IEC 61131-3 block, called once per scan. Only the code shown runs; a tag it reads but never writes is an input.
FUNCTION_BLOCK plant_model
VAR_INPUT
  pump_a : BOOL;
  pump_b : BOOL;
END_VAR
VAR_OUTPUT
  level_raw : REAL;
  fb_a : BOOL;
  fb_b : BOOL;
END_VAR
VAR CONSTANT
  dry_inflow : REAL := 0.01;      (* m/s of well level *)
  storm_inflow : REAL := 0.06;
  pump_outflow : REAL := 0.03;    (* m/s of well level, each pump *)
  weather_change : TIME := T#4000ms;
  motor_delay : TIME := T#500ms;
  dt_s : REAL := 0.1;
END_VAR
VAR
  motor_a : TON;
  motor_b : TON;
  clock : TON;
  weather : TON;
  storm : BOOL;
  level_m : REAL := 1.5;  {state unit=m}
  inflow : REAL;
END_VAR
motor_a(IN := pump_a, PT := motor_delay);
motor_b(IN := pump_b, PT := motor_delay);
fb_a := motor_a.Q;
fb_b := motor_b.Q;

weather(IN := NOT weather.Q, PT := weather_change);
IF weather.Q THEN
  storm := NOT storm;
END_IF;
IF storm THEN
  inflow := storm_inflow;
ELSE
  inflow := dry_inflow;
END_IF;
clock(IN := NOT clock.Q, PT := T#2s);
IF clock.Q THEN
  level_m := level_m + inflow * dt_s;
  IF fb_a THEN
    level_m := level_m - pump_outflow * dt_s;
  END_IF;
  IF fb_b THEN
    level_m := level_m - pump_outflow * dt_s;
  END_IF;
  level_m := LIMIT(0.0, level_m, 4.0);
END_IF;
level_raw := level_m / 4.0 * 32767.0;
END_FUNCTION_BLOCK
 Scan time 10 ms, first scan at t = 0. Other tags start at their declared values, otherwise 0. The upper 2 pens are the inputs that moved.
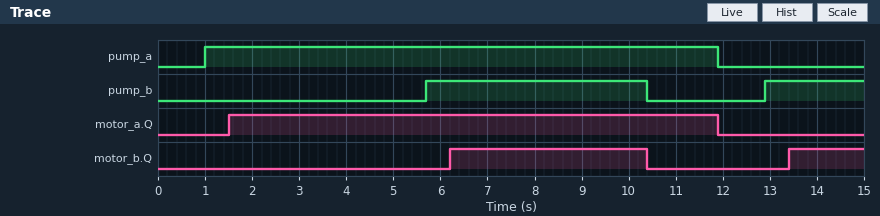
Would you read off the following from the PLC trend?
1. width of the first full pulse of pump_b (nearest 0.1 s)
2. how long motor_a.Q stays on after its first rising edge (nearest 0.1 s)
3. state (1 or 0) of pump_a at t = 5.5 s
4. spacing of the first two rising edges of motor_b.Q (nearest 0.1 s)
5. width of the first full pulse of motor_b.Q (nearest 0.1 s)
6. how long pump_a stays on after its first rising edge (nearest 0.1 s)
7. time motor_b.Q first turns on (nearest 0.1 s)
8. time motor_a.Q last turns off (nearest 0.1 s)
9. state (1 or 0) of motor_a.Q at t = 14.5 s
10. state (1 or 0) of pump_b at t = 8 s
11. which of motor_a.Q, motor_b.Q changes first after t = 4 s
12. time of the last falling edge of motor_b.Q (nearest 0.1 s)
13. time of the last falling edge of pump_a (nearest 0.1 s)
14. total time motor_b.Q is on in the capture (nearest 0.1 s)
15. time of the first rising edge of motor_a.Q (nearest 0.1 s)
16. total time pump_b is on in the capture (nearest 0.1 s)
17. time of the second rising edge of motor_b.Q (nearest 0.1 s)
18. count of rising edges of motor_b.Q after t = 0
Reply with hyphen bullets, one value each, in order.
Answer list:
- 4.7 s
- 10.4 s
- 1
- 7.2 s
- 4.2 s
- 10.9 s
- 6.2 s
- 11.9 s
- 0
- 1
- motor_b.Q
- 10.4 s
- 11.9 s
- 5.8 s
- 1.5 s
- 6.8 s
- 13.4 s
- 2
